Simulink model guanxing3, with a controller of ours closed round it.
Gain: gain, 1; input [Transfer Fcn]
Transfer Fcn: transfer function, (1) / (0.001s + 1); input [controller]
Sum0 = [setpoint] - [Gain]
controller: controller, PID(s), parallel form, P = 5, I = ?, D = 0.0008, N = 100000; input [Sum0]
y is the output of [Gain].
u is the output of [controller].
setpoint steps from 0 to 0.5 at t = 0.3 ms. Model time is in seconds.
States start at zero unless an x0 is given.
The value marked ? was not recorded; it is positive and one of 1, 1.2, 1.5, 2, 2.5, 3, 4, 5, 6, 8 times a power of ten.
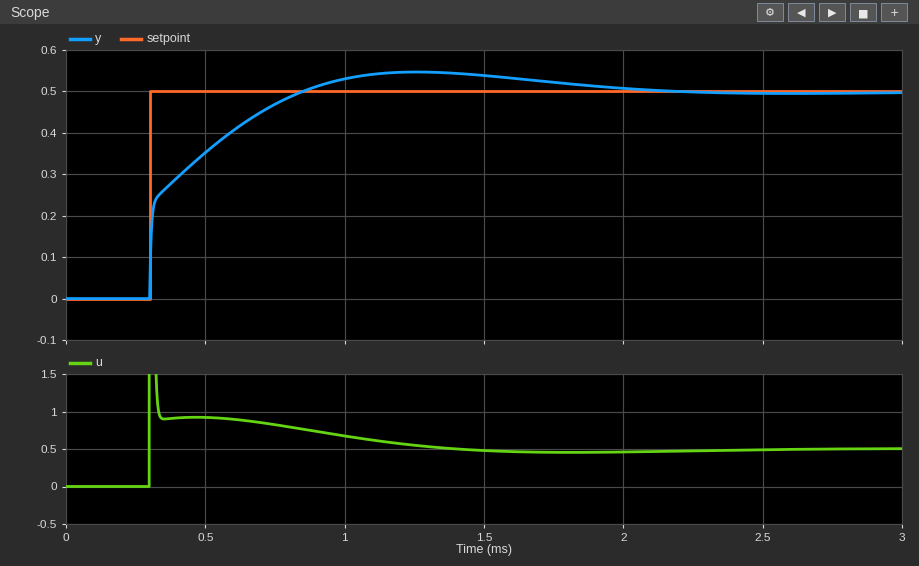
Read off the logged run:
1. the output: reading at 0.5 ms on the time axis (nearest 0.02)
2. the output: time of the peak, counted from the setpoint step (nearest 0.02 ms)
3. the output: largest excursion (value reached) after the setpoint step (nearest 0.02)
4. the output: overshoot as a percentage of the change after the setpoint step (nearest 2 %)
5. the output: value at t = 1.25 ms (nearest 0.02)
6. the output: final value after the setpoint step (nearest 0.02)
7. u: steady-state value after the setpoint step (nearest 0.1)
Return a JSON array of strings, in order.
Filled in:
["0.36", "0.96 ms", "0.54", "10 %", "0.54", "0.50", "0.5"]
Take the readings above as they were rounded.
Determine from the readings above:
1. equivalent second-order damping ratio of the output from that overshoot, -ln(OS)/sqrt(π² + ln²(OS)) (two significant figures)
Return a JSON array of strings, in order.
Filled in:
["0.59"]
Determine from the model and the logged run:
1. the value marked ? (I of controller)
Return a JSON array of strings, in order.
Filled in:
["15000"]
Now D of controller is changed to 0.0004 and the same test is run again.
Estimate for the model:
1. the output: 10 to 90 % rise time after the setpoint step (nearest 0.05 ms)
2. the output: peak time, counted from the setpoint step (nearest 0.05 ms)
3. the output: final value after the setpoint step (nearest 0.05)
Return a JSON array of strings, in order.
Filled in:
["0.35 ms", "0.80 ms", "0.50"]
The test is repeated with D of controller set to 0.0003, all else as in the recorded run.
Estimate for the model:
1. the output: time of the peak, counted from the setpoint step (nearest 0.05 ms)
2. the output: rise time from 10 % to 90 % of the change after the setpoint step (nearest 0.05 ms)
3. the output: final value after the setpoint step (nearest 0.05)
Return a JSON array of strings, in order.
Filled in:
["0.75 ms", "0.35 ms", "0.50"]
